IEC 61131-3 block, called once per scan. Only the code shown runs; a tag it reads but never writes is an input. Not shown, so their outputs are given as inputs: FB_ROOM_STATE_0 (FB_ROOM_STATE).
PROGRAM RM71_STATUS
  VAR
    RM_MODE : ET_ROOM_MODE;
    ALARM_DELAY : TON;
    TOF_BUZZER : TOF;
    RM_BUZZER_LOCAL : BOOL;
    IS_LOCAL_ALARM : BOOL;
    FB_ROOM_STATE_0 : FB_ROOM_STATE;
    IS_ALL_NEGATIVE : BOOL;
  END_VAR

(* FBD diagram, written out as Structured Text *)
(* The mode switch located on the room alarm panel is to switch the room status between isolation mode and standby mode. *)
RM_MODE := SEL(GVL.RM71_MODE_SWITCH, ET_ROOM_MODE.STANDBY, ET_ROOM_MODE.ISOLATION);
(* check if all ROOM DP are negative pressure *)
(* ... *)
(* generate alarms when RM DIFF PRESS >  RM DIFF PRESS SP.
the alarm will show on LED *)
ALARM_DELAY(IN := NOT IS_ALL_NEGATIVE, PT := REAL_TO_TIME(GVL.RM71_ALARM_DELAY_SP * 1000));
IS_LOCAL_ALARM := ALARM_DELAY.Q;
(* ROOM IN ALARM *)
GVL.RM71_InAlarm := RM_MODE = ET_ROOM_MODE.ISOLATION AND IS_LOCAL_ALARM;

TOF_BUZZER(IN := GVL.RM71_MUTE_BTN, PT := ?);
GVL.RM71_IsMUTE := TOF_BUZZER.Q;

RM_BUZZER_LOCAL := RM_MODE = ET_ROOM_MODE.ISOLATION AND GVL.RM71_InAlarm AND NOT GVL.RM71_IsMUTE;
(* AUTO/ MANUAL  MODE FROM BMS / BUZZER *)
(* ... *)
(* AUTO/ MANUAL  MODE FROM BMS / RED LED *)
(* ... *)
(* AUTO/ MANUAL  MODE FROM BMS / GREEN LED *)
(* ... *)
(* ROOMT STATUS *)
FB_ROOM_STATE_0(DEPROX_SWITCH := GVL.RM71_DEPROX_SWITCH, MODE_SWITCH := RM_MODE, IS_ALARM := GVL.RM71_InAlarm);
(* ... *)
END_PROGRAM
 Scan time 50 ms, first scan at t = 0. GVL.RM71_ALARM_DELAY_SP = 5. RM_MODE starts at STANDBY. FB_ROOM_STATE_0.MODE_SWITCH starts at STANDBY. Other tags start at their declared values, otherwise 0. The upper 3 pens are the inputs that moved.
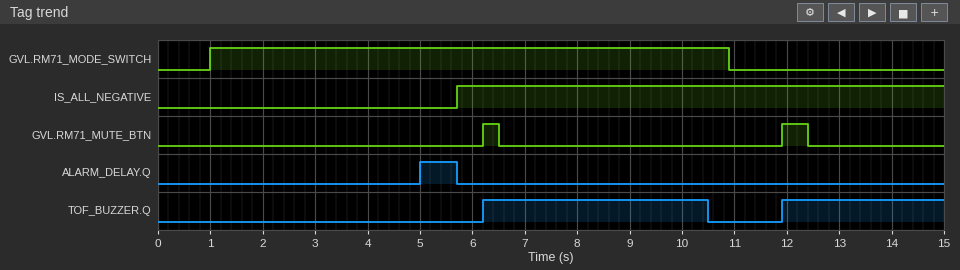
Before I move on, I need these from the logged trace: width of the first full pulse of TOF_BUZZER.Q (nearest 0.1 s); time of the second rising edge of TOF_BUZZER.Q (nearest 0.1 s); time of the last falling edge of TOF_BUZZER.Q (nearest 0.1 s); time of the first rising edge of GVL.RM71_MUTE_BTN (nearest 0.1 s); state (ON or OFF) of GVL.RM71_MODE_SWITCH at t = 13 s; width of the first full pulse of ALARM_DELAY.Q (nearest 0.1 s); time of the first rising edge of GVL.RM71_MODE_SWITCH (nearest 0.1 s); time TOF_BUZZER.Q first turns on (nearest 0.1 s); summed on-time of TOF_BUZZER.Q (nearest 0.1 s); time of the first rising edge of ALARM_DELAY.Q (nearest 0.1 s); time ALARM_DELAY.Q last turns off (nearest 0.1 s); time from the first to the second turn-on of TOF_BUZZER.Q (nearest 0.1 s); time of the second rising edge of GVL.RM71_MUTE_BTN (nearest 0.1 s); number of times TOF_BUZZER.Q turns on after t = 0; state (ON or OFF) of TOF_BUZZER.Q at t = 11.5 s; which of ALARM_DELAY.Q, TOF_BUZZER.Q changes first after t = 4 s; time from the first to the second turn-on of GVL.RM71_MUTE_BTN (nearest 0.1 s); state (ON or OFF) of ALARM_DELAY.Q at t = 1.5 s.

4.3 s
11.9 s
10.5 s
6.2 s
OFF
0.7 s
1.0 s
6.2 s
7.4 s
5.0 s
5.7 s
5.7 s
11.9 s
2
OFF
ALARM_DELAY.Q
5.7 s
OFF
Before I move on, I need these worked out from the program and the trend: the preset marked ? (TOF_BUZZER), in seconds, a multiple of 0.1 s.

4.0 s
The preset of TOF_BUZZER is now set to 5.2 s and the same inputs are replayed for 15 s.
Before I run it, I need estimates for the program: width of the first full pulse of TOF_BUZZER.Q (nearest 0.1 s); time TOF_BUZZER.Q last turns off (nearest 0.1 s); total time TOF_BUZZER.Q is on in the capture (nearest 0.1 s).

5.5 s
11.7 s
8.6 s
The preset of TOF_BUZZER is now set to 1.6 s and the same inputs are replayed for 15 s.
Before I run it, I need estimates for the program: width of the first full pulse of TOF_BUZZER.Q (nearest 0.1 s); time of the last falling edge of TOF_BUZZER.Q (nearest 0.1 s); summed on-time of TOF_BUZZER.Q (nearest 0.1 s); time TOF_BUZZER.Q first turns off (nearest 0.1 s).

1.9 s
14.0 s
4.0 s
8.1 s
